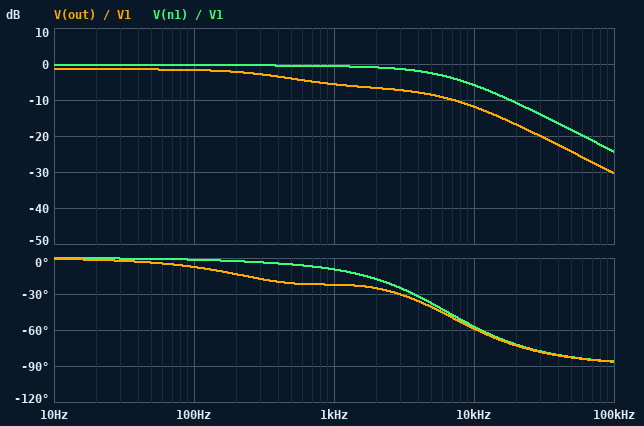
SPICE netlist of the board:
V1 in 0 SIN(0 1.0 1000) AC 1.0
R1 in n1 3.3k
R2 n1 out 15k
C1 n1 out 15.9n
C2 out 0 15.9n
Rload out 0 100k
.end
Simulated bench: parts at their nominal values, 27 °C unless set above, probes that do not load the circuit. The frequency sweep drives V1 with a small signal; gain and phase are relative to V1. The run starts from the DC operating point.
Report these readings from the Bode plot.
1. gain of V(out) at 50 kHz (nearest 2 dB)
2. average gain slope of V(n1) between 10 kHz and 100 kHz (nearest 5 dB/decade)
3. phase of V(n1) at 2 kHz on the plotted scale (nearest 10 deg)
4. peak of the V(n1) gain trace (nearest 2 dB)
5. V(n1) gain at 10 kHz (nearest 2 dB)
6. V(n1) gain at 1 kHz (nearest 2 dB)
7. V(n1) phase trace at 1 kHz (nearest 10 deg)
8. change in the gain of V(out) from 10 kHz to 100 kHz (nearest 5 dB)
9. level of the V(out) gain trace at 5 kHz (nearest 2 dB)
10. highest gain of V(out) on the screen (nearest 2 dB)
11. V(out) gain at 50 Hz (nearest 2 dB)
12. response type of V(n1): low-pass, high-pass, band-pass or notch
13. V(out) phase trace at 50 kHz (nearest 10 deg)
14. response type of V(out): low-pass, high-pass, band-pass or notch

-24 dB
-20 dB/decade
-20 deg
0 dB
-6 dB
0 dB
-10 deg
-20 dB
-8 dB
-2 dB
-2 dB
low-pass
-80 deg
low-pass
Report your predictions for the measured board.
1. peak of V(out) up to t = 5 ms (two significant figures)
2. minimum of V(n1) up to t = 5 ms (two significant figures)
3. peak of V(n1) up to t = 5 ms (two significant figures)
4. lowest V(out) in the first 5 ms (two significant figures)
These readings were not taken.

590 mV
-930 mV
940 mV
-520 mV
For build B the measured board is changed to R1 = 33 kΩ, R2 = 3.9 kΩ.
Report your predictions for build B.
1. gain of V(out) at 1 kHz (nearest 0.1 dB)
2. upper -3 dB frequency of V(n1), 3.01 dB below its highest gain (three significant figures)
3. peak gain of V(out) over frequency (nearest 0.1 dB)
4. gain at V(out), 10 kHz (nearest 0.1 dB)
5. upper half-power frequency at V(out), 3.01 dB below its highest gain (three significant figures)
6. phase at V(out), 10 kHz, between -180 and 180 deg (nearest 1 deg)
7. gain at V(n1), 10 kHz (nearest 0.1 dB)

-11.9 dB
390 Hz
-2.7 dB
-30.4 dB
368 Hz
-86 deg
-24.6 dB
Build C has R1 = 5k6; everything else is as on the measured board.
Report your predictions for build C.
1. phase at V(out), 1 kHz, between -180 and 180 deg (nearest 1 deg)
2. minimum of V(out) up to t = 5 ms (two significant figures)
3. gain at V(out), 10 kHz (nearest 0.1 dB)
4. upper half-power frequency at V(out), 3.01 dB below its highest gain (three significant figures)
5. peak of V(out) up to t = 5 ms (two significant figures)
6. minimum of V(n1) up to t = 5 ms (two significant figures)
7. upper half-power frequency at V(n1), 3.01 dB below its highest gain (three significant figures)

-28 deg
-490 mV
-15.6 dB
544 Hz
560 mV
-880 mV
3.51 kHz
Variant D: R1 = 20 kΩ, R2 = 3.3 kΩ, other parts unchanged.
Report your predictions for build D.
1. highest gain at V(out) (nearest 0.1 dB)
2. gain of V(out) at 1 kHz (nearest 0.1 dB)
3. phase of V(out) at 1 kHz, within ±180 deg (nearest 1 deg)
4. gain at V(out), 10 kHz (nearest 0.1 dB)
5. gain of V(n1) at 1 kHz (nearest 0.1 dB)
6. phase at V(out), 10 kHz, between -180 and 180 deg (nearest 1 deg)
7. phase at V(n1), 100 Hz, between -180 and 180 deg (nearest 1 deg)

-1.8 dB
-8.4 dB
-60 deg
-26.2 dB
-7.1 dB
-84 deg
-9 deg
